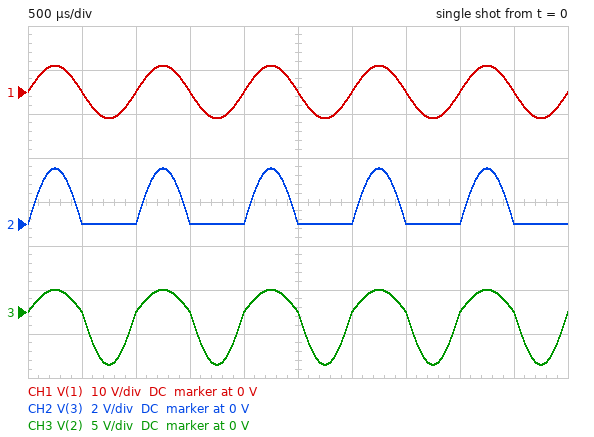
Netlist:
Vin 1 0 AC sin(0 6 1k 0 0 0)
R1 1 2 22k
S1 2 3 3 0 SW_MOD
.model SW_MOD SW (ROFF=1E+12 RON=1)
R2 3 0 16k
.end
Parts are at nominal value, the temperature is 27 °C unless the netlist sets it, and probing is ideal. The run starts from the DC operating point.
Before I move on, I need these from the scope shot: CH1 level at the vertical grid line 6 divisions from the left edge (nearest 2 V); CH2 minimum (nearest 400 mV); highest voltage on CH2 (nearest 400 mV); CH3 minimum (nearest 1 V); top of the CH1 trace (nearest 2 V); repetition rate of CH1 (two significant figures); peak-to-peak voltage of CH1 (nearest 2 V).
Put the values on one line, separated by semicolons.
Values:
0 V; 0 V; 2.4 V; -6 V; 6 V; 1.0 kHz; 12 V
